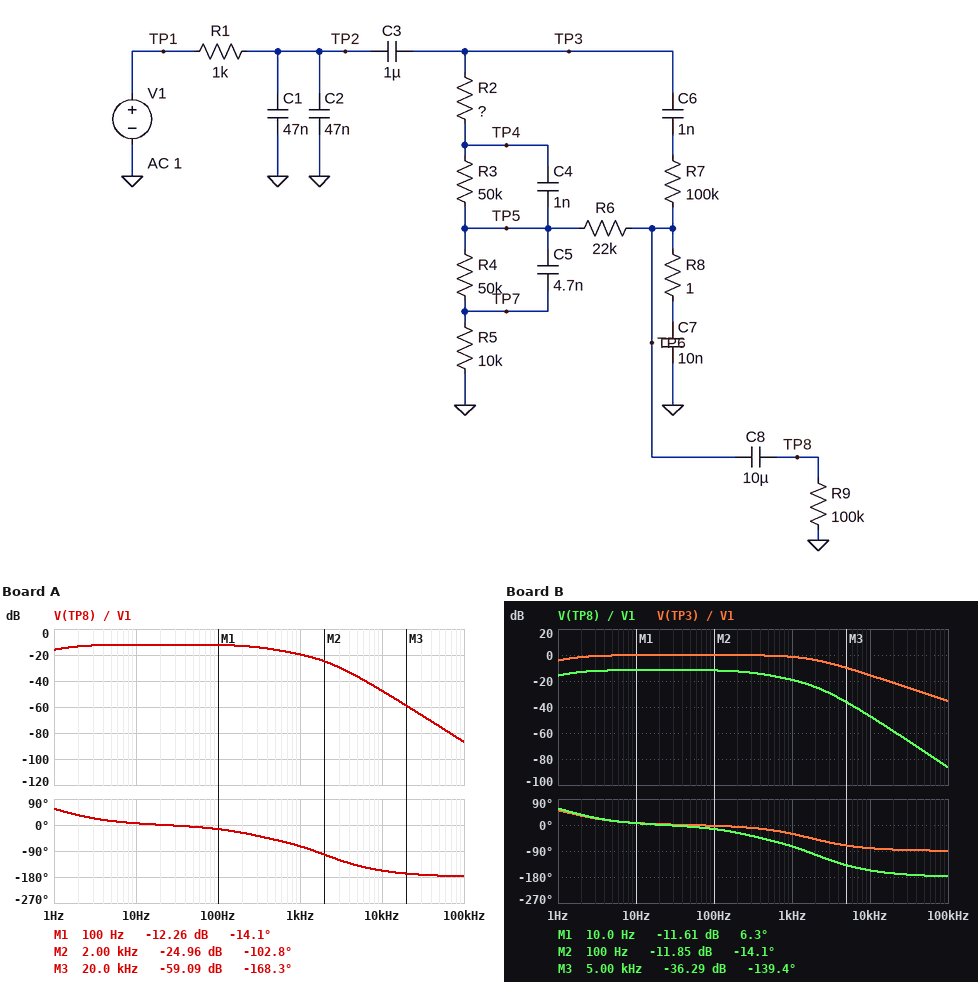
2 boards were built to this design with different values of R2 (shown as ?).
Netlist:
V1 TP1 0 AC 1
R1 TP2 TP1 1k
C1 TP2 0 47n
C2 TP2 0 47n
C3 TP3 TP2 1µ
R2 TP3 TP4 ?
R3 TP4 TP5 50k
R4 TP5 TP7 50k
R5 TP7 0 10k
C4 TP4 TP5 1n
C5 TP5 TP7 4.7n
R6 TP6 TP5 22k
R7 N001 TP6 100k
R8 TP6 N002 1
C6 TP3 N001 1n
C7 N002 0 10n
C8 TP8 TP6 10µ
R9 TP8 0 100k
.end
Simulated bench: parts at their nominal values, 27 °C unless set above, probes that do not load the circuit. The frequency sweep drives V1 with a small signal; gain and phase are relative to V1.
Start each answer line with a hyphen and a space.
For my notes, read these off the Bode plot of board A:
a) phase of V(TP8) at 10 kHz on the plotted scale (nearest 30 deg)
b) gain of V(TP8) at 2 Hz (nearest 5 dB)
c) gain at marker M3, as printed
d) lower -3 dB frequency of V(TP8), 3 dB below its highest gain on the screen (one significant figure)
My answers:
- -150 deg
- -15 dB
- -59.09 dB
- 1 Hz
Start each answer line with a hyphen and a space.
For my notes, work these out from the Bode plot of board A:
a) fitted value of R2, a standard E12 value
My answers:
- 39 kΩ
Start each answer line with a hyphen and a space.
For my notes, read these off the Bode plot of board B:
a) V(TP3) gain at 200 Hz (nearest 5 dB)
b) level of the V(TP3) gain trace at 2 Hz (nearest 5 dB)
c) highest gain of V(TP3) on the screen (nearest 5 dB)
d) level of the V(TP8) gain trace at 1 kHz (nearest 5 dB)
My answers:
- 0 dB
- 0 dB
- 0 dB
- -20 dB
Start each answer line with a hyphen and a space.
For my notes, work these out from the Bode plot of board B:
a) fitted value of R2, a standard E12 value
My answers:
- 33 kΩ
